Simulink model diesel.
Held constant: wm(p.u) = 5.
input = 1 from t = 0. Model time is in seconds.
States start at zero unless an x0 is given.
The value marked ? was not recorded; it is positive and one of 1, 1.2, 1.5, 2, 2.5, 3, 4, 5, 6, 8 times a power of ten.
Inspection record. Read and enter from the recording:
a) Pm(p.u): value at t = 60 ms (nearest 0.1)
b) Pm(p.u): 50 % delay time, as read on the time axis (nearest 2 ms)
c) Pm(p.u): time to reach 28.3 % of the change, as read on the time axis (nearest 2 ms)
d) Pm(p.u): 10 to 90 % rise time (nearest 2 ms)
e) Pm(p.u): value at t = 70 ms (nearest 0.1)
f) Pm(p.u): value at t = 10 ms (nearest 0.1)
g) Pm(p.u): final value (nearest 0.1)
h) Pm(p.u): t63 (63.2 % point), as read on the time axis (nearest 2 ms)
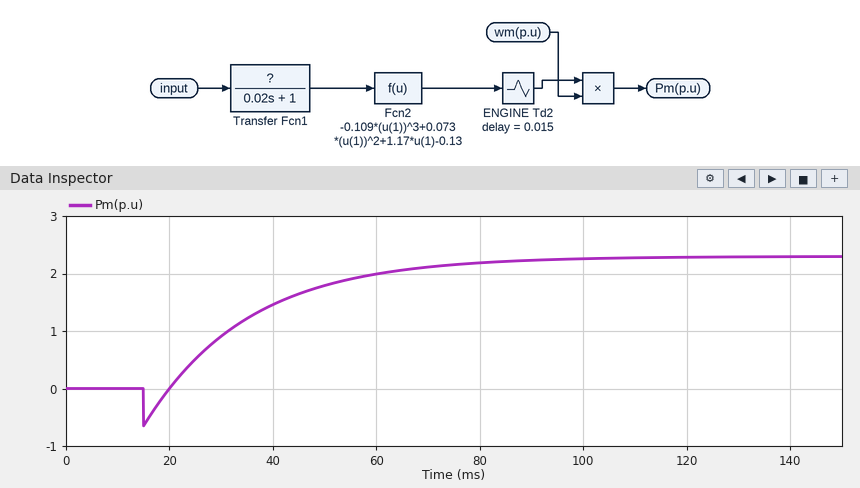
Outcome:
2.0
34 ms
26 ms
44 ms
2.1
0.0
2.3
40 ms
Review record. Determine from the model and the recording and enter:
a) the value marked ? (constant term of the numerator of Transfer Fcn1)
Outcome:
0.5
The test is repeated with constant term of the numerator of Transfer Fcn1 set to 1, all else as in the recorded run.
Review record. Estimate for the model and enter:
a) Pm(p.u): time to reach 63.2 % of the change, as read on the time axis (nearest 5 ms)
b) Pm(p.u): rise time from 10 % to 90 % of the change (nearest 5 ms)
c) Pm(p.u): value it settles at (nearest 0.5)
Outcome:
35 ms
40 ms
5.0
